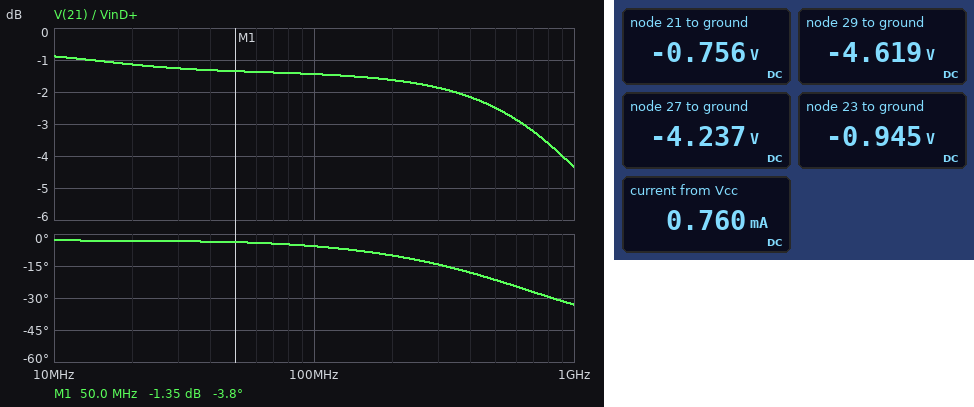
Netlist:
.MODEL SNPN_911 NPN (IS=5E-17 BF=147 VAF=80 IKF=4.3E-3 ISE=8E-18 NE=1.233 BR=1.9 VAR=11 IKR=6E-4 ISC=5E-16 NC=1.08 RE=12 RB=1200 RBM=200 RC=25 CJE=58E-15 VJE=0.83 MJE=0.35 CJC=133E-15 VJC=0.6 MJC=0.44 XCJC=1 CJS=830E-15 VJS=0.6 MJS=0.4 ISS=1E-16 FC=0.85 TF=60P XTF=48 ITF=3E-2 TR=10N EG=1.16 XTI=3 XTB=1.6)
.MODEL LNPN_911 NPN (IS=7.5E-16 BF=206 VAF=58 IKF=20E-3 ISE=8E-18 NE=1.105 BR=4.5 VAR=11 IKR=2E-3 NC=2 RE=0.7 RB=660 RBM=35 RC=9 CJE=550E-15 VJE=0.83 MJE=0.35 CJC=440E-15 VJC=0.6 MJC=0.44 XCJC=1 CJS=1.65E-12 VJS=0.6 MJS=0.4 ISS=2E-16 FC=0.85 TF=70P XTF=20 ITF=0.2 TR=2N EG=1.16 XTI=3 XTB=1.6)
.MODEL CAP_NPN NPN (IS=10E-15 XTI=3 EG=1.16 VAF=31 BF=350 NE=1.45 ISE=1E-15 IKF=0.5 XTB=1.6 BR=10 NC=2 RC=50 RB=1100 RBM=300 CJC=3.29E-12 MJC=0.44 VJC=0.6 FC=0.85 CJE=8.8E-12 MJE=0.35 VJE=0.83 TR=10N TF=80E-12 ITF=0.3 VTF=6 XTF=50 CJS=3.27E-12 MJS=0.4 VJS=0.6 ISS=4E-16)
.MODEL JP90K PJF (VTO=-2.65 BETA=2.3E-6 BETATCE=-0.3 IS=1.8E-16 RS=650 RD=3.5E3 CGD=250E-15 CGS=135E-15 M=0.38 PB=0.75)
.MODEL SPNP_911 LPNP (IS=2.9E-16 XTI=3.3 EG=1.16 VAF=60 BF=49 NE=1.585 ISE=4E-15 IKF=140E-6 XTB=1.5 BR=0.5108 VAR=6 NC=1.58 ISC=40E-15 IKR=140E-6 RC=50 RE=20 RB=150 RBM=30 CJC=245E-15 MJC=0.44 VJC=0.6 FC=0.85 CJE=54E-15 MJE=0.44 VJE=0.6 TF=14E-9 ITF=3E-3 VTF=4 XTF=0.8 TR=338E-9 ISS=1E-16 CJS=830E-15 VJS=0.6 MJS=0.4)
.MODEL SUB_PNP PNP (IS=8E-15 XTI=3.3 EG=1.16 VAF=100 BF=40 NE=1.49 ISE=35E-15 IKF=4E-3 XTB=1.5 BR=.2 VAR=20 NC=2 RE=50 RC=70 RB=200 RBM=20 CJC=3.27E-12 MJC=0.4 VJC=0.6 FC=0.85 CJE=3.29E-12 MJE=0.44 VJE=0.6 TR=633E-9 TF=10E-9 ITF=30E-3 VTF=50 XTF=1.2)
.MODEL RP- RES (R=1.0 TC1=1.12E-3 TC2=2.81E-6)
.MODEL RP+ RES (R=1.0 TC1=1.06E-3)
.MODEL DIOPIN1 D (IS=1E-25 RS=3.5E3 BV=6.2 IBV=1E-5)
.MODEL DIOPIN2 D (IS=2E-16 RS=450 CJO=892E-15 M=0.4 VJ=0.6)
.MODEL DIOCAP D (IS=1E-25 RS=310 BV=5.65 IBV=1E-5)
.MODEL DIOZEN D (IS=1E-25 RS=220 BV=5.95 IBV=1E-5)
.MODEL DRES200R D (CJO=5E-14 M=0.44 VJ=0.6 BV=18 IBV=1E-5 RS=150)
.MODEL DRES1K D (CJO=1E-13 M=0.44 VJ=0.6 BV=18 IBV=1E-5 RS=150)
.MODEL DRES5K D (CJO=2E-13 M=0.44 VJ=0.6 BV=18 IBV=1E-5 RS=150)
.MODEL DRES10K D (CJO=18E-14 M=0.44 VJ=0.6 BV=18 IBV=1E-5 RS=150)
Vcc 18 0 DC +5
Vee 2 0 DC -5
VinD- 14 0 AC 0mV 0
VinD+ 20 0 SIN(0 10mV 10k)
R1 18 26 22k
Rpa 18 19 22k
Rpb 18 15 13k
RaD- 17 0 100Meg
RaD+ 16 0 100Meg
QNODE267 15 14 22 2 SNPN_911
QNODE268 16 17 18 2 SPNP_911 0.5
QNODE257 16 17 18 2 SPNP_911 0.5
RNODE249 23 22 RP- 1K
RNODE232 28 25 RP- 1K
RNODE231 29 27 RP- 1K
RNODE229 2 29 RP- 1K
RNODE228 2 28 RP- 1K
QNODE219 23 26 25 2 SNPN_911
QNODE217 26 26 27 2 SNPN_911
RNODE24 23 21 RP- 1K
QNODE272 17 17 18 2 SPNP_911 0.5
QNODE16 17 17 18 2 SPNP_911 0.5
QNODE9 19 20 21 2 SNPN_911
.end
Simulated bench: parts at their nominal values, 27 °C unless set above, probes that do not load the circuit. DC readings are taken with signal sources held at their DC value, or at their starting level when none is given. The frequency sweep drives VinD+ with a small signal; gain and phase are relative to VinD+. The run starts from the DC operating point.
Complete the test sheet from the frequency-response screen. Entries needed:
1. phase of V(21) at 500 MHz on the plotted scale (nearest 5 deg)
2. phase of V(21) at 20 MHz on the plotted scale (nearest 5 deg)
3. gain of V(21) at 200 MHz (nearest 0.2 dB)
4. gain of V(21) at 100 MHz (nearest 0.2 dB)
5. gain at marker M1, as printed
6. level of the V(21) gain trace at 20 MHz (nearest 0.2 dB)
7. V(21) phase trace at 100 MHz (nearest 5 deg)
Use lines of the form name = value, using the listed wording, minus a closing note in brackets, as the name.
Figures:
phase of V(21) at 500 MHz on the plotted scale = -20 deg
phase of V(21) at 20 MHz on the plotted scale = -5 deg
gain of V(21) at 200 MHz = -1.6 dB
gain of V(21) at 100 MHz = -1.4 dB
gain at marker M1, as printed = -1.35 dB
level of the V(21) gain trace at 20 MHz = -1.2 dB
V(21) phase trace at 100 MHz = -5 deg
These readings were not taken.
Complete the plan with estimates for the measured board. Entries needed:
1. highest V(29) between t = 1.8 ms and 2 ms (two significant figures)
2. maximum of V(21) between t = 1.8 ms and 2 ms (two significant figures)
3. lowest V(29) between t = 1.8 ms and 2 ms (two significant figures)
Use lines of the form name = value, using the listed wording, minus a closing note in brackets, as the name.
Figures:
highest V(29) between t = 1.8 ms and 2 ms = -4.6 V
maximum of V(21) between t = 1.8 ms and 2 ms = -750 mV
lowest V(29) between t = 1.8 ms and 2 ms = -4.6 V
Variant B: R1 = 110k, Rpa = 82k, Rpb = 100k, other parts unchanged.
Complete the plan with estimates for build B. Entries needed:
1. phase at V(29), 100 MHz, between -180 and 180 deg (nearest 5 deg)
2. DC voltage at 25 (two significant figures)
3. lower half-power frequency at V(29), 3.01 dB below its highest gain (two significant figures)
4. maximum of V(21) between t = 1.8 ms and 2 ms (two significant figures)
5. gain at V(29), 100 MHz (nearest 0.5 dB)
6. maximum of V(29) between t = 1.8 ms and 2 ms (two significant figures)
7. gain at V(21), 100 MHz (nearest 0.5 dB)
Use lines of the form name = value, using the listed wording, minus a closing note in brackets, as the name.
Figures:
phase at V(29), 100 MHz, between -180 and 180 deg = 25 deg
DC voltage at 25 = -4.8 V
lower half-power frequency at V(29), 3.01 dB below its highest gain = 67 MHz
maximum of V(21) between t = 1.8 ms and 2 ms = -700 mV
gain at V(29), 100 MHz = -38.5 dB
maximum of V(29) between t = 1.8 ms and 2 ms = -4.9 V
gain at V(21), 100 MHz = -2.5 dB
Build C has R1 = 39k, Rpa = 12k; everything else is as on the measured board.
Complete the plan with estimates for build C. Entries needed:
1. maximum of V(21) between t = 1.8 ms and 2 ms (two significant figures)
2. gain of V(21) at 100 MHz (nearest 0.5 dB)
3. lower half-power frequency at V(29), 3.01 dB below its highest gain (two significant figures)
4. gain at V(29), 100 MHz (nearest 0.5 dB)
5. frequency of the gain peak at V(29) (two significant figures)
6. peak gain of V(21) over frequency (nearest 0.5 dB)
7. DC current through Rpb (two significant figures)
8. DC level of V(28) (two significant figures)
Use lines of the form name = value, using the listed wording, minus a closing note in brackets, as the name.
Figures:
maximum of V(21) between t = 1.8 ms and 2 ms = -730 mV
gain of V(21) at 100 MHz = -1.5 dB
lower half-power frequency at V(29), 3.01 dB below its highest gain = 82 MHz
gain at V(29), 100 MHz = -37.5 dB
frequency of the gain peak at V(29) = 230 MHz
peak gain of V(21) over frequency = -1.0 dB
DC current through Rpb = 110 µA
DC level of V(28) = -4.8 V
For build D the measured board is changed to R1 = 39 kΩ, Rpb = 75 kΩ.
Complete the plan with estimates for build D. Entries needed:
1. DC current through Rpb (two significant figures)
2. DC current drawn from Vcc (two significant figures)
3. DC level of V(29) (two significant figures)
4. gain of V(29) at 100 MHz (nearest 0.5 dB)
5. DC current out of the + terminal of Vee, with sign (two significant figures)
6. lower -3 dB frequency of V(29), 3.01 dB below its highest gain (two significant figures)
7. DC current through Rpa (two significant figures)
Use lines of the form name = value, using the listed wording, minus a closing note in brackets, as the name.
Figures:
DC current through Rpb = 76 µA
DC current drawn from Vcc = 420 µA
DC level of V(29) = -4.8 V
gain of V(29) at 100 MHz = -36.0 dB
DC current out of the + terminal of Vee, with sign = -450 µA
lower -3 dB frequency of V(29), 3.01 dB below its highest gain = 73 MHz
DC current through Rpa = 120 µA
